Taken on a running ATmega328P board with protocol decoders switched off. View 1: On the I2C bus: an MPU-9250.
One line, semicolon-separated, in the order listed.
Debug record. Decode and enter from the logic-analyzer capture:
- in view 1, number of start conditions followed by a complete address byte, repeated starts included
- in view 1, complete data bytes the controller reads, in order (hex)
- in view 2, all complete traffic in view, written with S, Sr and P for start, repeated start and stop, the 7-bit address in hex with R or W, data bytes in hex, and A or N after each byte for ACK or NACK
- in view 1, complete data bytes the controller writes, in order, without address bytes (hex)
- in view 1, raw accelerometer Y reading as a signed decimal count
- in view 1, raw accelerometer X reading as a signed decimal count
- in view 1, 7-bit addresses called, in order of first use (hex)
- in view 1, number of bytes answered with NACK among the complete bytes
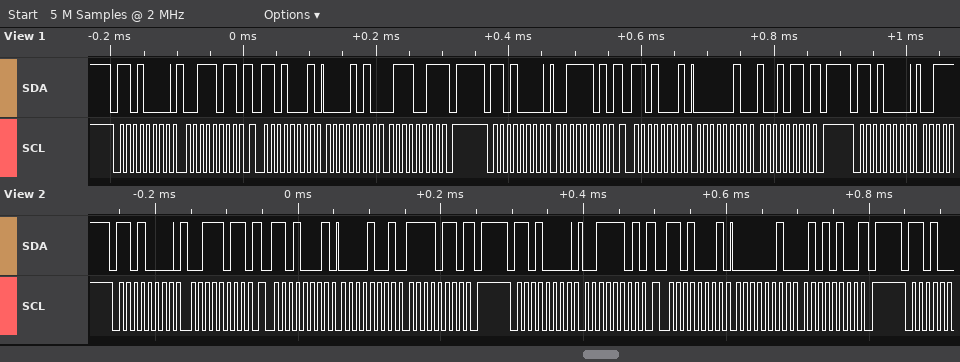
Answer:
5; 0A 73 02 96; S 68W A 3B A Sr 68R A 09 A F6 N P S 68W A 3D A Sr 68R A 02 A 54 N P; 3B 3D; 662; 2675; 0x68; 2
